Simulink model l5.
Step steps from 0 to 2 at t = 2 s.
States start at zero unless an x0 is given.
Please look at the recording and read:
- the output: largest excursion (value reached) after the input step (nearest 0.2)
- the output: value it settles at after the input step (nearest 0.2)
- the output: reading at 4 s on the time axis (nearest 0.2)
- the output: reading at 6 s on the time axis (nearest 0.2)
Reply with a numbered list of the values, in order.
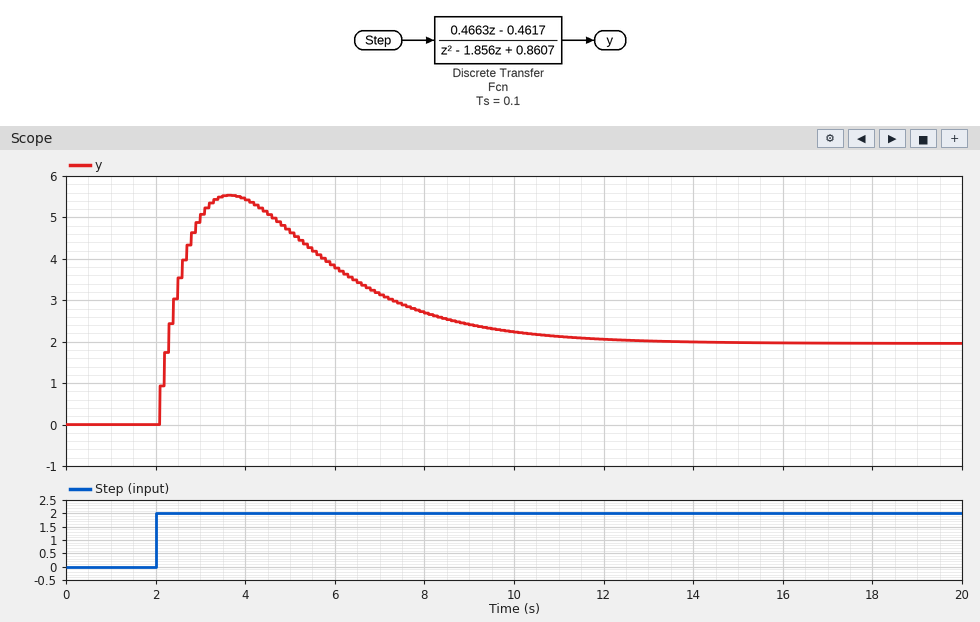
1. 5.6
2. 2.0
3. 5.4
4. 3.8
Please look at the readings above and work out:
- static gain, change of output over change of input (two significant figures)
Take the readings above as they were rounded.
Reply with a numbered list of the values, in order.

1. 1.0
